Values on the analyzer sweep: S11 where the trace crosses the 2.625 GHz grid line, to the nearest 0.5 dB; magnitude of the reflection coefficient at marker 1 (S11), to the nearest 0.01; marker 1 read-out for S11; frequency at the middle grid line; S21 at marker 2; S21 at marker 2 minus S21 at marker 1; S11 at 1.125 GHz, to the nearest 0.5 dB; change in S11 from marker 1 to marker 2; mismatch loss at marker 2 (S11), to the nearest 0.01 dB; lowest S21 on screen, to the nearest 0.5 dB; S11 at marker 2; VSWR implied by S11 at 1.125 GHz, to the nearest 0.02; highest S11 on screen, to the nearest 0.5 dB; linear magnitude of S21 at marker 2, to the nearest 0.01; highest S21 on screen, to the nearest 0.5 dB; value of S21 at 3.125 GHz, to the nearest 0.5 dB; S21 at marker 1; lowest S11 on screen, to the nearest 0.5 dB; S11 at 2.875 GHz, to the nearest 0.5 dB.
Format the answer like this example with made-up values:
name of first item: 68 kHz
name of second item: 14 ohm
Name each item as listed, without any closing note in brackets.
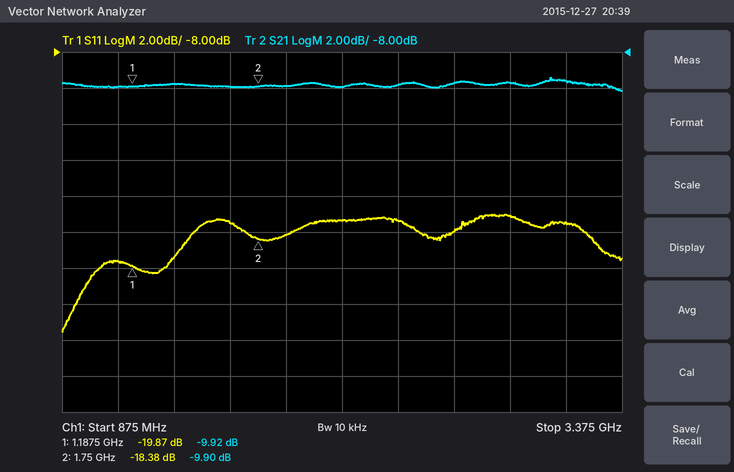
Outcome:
S11 where the trace crosses the 2.625 GHz grid line, to the nearest 0.5 dB: -18.0 dB
magnitude of the reflection coefficient at marker 1 (S11), to the nearest 0.01: 0.10
marker 1 read-out for S11: -19.87 dB
frequency at the middle grid line: 2.125 GHz
S21 at marker 2: -9.90 dB
S21 at marker 2 minus S21 at marker 1: 0.02 dB
S11 at 1.125 GHz, to the nearest 0.5 dB: -19.5 dB
change in S11 from marker 1 to marker 2: 1.49 dB
mismatch loss at marker 2 (S11), to the nearest 0.01 dB: 0.06 dB
lowest S21 on screen, to the nearest 0.5 dB: -10.0 dB
S11 at marker 2: -18.38 dB
VSWR implied by S11 at 1.125 GHz, to the nearest 0.02: 1.24
highest S11 on screen, to the nearest 0.5 dB: -17.0 dB
linear magnitude of S21 at marker 2, to the nearest 0.01: 0.32
highest S21 on screen, to the nearest 0.5 dB: -9.5 dB
value of S21 at 3.125 GHz, to the nearest 0.5 dB: -9.5 dB
S21 at marker 1: -9.92 dB
lowest S11 on screen, to the nearest 0.5 dB: -23.5 dB
S11 at 2.875 GHz, to the nearest 0.5 dB: -17.0 dB
